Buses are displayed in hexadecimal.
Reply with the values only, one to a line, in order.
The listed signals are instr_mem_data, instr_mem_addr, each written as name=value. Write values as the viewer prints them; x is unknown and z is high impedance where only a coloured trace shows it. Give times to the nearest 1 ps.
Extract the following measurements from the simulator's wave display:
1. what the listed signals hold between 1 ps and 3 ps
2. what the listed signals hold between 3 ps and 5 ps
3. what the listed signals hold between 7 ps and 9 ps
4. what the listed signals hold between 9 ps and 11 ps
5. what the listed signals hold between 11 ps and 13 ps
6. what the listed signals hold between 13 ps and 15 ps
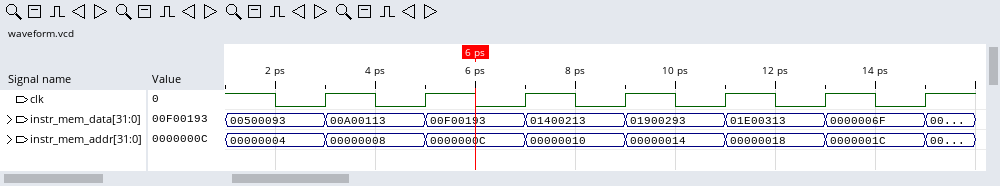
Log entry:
instr_mem_data=00500093, instr_mem_addr=00000004
instr_mem_data=00A00113, instr_mem_addr=00000008
instr_mem_data=01400213, instr_mem_addr=00000010
instr_mem_data=01900293, instr_mem_addr=00000014
instr_mem_data=01E00313, instr_mem_addr=00000018
instr_mem_data=0000006F, instr_mem_addr=0000001C
